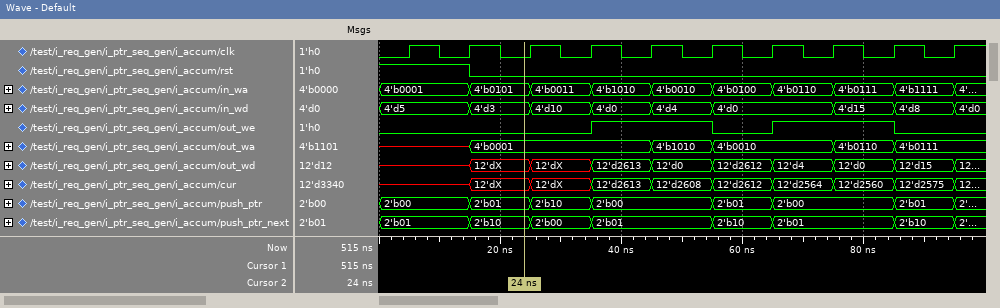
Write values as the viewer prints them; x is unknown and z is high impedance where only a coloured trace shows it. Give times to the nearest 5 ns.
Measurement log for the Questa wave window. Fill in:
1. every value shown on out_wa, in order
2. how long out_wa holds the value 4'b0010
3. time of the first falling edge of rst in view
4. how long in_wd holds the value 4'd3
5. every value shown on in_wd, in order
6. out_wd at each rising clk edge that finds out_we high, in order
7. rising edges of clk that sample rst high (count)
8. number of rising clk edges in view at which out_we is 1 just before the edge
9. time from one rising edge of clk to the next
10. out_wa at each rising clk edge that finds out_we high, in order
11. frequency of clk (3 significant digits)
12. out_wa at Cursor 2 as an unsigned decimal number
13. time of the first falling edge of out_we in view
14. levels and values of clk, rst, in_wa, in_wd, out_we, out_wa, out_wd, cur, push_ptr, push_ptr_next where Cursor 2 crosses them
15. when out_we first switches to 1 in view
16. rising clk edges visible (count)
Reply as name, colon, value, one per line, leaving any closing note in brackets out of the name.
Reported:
every value shown on out_wa, in order: x, 4'b0001, 4'b1010, 4'b0010, 4'b0110, 4'b0111
how long out_wa holds the value 4'b0010: 20 ns
time of the first falling edge of rst in view: 15 ns
how long in_wd holds the value 4'd3: 10 ns
every value shown on in_wd, in order: 4'd5, 4'd3, 4'd10, 4'd0, 4'd4, 4'd0, 4'd15, 4'd8, 4'd0
out_wd at each rising clk edge that finds out_we high, in order: 12'd2613, 12'd0, 12'd4, 12'd0
rising edges of clk that sample rst high: 2
number of rising clk edges in view at which out_we is 1 just before the edge: 4
time from one rising edge of clk to the next: 10 ns
out_wa at each rising clk edge that finds out_we high, in order: 4'b0001, 4'b1010, 4'b0010, 4'b0110
frequency of clk: 100 MHz
out_wa at Cursor 2 as an unsigned decimal number: 1
time of the first falling edge of out_we in view: 55 ns
levels and values of clk, rst, in_wa, in_wd, out_we, out_wa, out_wd, cur, push_ptr, push_ptr_next where Cursor 2 crosses them: clk=0, rst=0, in_wa=4'b0101, in_wd=4'd3, out_we=0, out_wa=4'b0001, out_wd=12'dX, cur=12'dX, push_ptr=2'b01, push_ptr_next=2'b10
when out_we first switches to 1 in view: 35 ns
rising clk edges visible: 10
